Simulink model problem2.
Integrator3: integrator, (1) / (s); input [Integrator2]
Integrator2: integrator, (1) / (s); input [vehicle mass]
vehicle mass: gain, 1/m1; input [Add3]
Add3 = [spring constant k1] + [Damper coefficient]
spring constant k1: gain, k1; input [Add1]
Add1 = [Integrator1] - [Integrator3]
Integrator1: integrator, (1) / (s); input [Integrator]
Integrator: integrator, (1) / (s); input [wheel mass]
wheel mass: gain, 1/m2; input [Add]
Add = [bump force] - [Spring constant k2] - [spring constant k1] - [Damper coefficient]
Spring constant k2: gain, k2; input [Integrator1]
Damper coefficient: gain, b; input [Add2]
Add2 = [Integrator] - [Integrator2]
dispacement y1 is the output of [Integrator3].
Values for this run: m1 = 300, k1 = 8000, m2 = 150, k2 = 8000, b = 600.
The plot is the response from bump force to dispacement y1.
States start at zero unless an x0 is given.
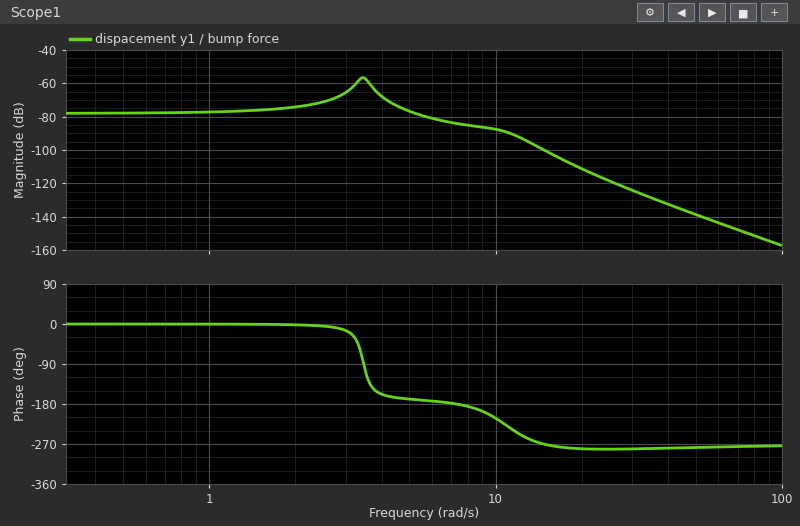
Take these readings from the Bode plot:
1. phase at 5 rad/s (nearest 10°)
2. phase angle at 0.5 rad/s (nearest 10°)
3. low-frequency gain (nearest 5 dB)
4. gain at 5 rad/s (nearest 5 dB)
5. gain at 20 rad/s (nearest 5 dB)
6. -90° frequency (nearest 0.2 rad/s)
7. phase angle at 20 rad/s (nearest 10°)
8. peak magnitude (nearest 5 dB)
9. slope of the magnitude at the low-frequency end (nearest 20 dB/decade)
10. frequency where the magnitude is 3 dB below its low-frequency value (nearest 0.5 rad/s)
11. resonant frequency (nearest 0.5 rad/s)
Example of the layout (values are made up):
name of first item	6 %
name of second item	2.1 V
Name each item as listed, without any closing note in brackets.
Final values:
phase at 5 rad/s	-170°
phase angle at 0.5 rad/s	0°
low-frequency gain	-80 dB
gain at 5 rad/s	-75 dB
gain at 20 rad/s	-110 dB
-90° frequency	3.4 rad/s
phase angle at 20 rad/s	-280°
peak magnitude	-55 dB
slope of the magnitude at the low-frequency end	0 dB/decade
frequency where the magnitude is 3 dB below its low-frequency value	6.0 rad/s
resonant frequency	3.5 rad/s
